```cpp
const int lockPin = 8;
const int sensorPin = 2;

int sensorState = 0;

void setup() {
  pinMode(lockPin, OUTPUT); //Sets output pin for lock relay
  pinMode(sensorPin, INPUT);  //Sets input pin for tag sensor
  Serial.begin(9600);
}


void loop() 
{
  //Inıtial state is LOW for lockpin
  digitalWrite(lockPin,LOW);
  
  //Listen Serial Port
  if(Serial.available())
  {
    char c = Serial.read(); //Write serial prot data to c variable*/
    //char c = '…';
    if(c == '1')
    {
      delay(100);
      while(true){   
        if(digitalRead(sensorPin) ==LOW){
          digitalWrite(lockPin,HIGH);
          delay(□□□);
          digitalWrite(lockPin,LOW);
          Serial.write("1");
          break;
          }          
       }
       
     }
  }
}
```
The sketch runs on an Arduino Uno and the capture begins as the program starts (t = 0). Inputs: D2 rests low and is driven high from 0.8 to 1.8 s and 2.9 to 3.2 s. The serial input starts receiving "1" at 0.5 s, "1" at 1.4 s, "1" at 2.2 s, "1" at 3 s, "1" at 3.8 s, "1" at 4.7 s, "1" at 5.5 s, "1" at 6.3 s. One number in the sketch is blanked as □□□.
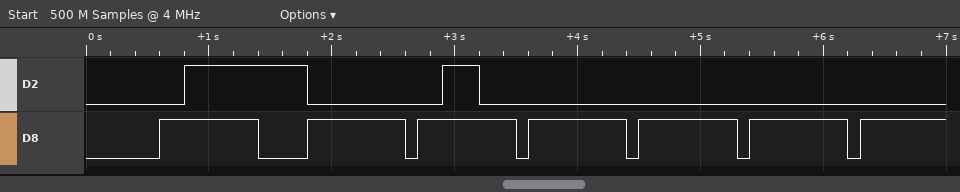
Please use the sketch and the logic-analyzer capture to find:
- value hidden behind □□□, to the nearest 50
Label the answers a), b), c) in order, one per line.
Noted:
a) 800
